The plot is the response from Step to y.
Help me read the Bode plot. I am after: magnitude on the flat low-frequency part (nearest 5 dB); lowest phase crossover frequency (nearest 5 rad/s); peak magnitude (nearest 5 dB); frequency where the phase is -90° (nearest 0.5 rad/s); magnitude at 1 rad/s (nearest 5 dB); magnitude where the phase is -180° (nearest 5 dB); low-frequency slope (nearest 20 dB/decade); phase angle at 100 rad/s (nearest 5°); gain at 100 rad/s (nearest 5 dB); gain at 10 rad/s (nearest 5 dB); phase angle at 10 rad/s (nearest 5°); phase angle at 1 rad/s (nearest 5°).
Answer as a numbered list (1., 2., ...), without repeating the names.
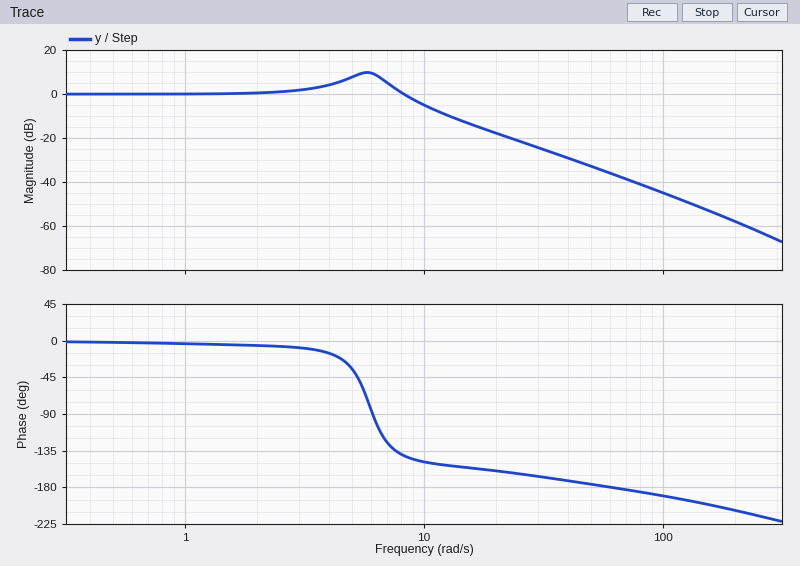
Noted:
1. 0 dB
2. 60 rad/s
3. 10 dB
4. 6.0 rad/s
5. 0 dB
6. -35 dB
7. 0 dB/decade
8. -190°
9. -45 dB
10. -5 dB
11. -150°
12. -5°
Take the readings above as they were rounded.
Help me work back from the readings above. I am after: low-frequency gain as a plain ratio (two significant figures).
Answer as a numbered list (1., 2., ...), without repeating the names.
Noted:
1. 1.0
